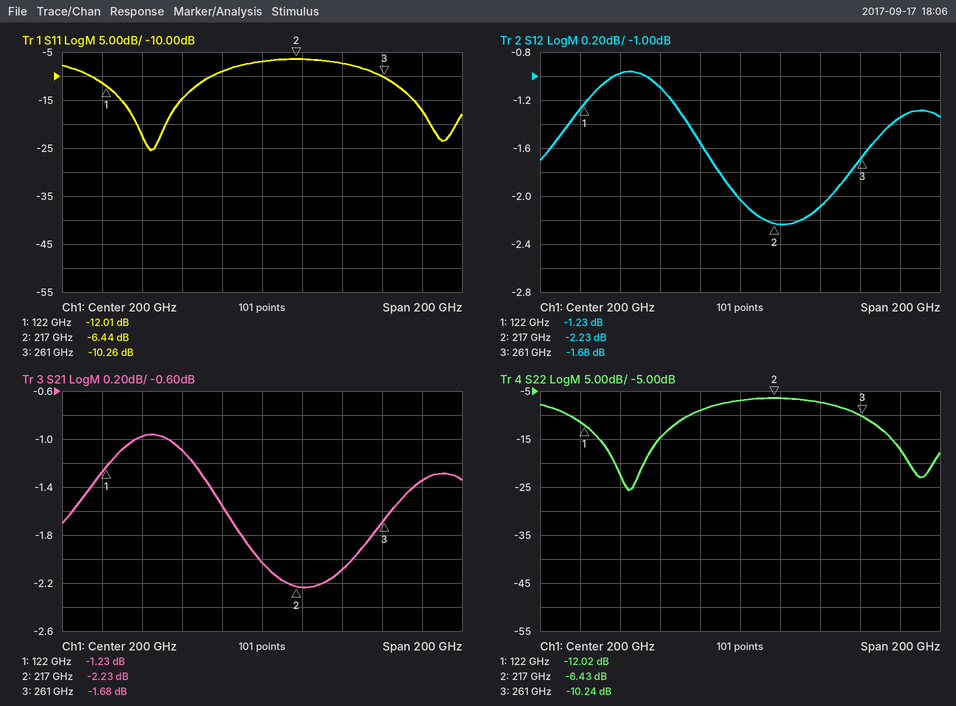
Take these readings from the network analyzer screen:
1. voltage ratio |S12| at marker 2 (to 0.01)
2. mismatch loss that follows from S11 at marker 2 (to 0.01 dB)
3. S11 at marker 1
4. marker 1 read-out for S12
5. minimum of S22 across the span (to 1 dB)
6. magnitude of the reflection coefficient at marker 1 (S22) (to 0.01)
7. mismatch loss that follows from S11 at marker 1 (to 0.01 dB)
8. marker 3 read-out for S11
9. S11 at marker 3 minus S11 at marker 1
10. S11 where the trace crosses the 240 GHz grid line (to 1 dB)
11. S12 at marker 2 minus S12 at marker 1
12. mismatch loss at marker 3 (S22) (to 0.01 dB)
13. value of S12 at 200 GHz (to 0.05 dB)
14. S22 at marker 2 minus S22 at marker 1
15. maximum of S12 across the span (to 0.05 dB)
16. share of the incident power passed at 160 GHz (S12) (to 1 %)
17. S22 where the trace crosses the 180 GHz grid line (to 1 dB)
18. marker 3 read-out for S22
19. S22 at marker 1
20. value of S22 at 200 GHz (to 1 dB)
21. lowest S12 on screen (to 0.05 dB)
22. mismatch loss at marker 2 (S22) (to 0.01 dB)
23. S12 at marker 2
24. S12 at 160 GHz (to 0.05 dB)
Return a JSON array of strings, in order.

["0.77", "1.12 dB", "-12.01 dB", "-1.23 dB", "-26 dB", "0.25", "0.28 dB", "-10.26 dB", "1.75 dB", "-7 dB", "-1.00 dB", "0.43 dB", "-2.05 dB", "5.59 dB", "-0.95 dB", "78 %", "-9 dB", "-10.24 dB", "-12.02 dB", "-7 dB", "-2.25 dB", "1.12 dB", "-2.23 dB", "-1.10 dB"]
